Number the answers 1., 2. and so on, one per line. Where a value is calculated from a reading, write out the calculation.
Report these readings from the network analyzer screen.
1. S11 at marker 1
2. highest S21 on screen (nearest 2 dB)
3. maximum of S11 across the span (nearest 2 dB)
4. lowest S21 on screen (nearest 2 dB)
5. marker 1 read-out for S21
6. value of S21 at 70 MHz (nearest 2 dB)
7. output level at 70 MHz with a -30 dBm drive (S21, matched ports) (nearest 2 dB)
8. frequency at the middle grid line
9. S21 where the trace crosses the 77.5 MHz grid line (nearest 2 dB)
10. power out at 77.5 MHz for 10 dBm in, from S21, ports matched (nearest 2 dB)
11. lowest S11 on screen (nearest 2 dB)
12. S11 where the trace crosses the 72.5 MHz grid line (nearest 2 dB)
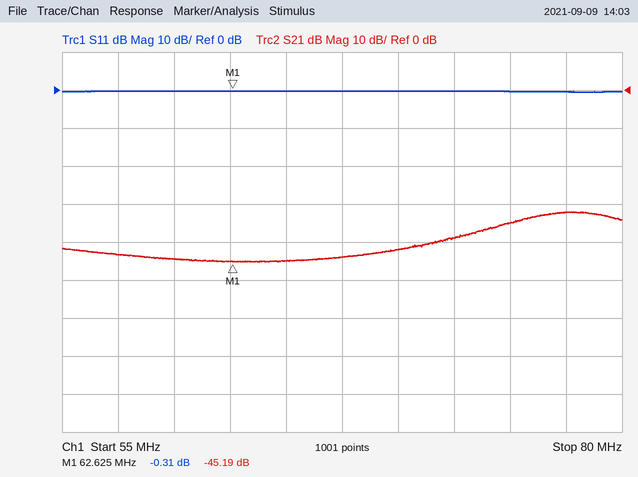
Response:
1. -0.31 dB
2. -32 dB
3. 0 dB
4. -46 dB
5. -45.19 dB
6. -42 dB
7. -30 dBm + (-42 dB) = -72 dBm
8. 67.5 MHz
9. -32 dB
10. 10 dBm + (-32 dB) = -22 dBm
11. 0 dB
12. 0 dB
